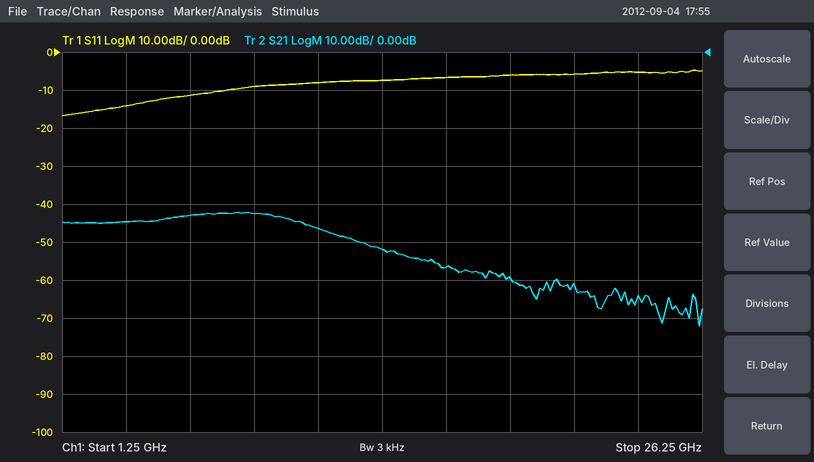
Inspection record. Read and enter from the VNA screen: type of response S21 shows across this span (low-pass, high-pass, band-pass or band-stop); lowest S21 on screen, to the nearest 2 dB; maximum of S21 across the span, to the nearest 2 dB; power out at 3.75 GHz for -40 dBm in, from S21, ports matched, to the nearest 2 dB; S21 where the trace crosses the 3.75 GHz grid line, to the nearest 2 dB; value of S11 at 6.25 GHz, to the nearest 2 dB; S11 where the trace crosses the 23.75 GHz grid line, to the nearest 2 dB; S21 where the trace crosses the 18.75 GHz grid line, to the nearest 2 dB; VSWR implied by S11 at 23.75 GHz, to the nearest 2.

low-pass
-72 dB
-42 dB
-84 dBm
-44 dB
-12 dB
-6 dB
-60 dB
4
